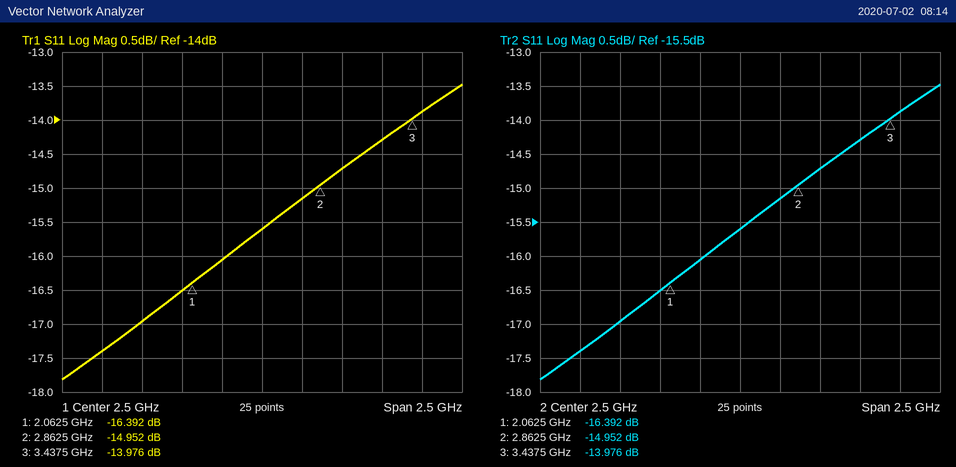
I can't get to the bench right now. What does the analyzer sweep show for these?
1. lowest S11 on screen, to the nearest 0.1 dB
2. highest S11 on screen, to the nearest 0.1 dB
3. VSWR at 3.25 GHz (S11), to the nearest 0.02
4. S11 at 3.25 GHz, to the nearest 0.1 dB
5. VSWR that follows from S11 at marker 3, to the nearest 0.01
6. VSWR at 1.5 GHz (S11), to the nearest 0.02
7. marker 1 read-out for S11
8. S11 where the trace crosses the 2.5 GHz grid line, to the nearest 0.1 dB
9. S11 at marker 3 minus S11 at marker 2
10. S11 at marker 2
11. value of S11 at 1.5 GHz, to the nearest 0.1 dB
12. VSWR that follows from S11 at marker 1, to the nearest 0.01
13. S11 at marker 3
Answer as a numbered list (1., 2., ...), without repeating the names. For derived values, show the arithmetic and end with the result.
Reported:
1. -17.8 dB
2. -13.5 dB
3. |Γ| = 10^(-14.3/20) = 0.1928; VSWR = (1 + 0.1928)/(1 − 0.1928) ≈ 1.48
4. -14.3 dB
5. (1 + 0.2001)/(1 − 0.2001) ≈ 1.50
6. |Γ| = 10^(-17.4/20) = 0.1349; VSWR = (1 + 0.1349)/(1 − 0.1349) ≈ 1.31, so 1.32 to the nearest 0.02
7. -16.392 dB
8. -15.6 dB
9. -13.976 − (-14.952) = 0.976 dB
10. -14.952 dB
11. -17.4 dB
12. (1 + 0.1515)/(1 − 0.1515) ≈ 1.36
13. -13.976 dB
